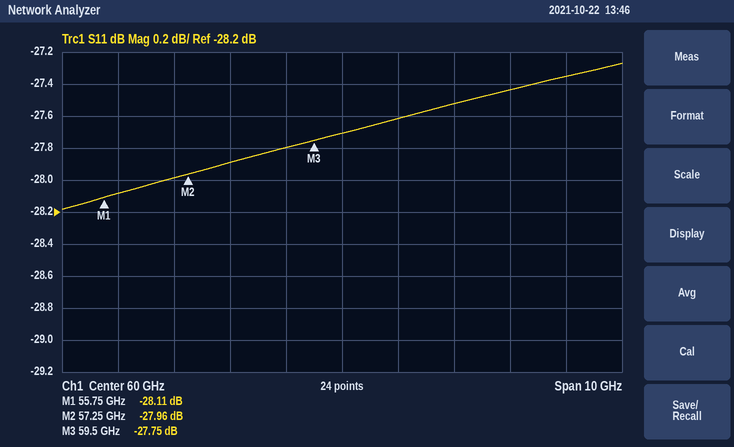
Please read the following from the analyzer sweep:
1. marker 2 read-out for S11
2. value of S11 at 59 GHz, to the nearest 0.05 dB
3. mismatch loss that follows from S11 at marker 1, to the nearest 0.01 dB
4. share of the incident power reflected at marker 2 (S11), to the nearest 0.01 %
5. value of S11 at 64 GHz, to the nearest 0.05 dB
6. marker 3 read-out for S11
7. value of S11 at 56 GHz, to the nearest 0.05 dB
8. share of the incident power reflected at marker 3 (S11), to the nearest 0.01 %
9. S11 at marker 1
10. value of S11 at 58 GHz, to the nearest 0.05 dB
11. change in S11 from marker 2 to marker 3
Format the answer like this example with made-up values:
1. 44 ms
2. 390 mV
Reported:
1. -27.96 dB
2. -27.80 dB
3. 0.01 dB
4. 0.16 %
5. -27.35 dB
6. -27.75 dB
7. -28.10 dB
8. 0.17 %
9. -28.11 dB
10. -27.90 dB
11. 0.21 dB
